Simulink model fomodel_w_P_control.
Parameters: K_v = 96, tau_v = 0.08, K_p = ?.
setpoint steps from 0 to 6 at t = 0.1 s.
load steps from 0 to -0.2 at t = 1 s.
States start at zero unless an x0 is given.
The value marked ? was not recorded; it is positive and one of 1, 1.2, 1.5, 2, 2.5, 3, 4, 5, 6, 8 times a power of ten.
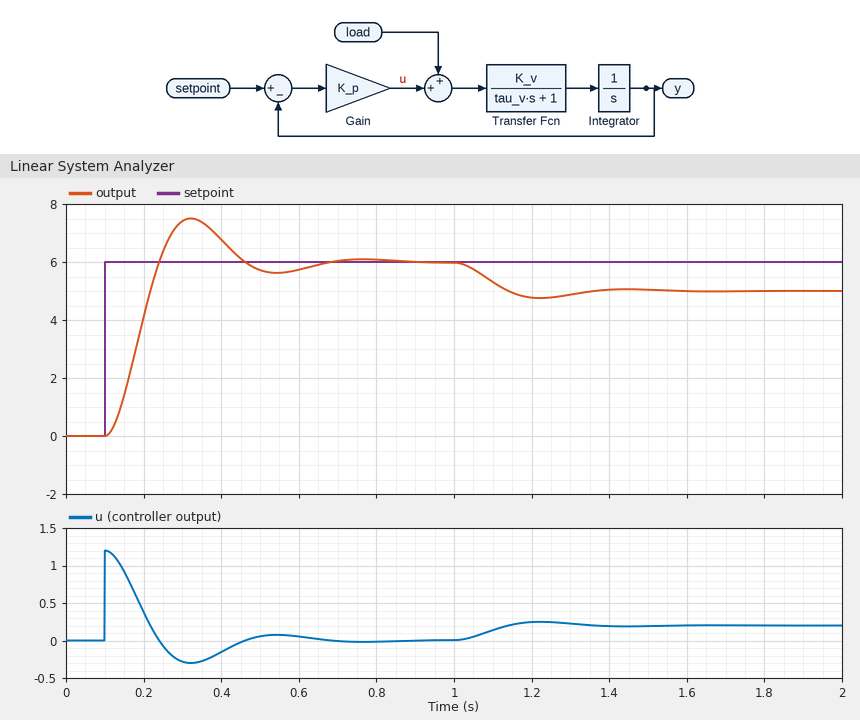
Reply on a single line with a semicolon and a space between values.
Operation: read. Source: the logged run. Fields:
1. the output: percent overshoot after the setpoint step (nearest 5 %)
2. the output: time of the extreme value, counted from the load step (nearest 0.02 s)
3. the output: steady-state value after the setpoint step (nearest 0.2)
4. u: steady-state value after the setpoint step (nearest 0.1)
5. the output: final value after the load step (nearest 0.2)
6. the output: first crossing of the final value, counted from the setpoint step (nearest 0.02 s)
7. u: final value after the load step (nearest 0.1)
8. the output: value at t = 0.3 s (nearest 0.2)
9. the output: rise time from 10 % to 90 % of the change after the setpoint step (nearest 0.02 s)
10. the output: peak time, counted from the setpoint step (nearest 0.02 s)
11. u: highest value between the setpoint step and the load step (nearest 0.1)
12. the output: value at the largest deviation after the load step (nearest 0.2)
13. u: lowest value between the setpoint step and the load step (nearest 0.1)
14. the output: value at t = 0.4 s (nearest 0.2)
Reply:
25 %; 0.22 s; 6.0; 0.0; 5.0; 0.14 s; 0.2; 7.4; 0.10 s; 0.22 s; 1.2; 4.8; -0.3; 6.8
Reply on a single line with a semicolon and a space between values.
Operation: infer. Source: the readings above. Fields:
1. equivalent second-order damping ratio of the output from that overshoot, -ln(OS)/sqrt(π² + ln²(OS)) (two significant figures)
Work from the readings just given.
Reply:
0.40
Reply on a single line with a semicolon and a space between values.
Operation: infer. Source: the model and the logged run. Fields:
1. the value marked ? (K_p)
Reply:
0.2
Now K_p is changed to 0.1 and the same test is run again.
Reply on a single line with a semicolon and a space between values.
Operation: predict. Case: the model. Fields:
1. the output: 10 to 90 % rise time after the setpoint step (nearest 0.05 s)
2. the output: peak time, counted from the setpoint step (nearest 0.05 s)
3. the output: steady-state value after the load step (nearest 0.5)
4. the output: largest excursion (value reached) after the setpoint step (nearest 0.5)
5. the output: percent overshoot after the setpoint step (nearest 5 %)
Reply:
0.15 s; 0.35 s; 4.0; 6.5; 10 %
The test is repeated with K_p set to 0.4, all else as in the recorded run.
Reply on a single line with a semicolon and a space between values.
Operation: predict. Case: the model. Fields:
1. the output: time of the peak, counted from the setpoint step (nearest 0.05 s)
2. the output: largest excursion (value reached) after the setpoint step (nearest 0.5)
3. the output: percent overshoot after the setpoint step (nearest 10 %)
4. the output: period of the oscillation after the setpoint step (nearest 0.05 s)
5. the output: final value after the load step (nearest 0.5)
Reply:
0.15 s; 8.5; 40 %; 0.30 s; 5.5
